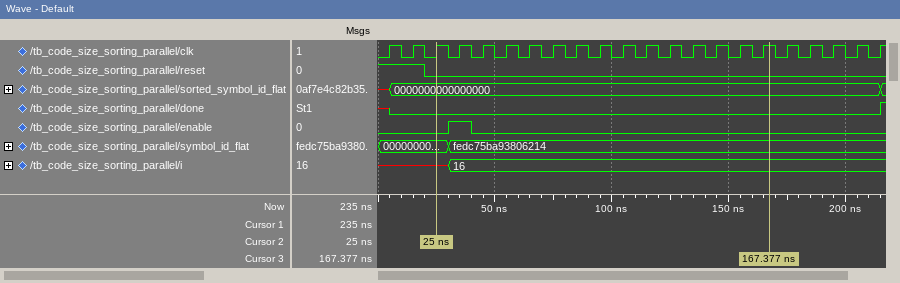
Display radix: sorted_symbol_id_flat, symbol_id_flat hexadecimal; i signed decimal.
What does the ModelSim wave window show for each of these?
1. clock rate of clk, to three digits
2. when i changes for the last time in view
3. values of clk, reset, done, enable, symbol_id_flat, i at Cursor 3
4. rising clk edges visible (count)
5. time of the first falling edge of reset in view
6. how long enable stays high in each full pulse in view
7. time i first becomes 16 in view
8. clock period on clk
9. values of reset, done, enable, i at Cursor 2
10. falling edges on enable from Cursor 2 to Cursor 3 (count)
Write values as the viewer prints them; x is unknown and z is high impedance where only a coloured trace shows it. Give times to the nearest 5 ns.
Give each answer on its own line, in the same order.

100 MHz
30 ns
clk=1, reset=0, done=0, enable=0, symbol_id_flat=fedc75ba93806214, i=16
22
20 ns
10 ns
30 ns
10 ns
reset=0, done=0, enable=0, i=x
1
